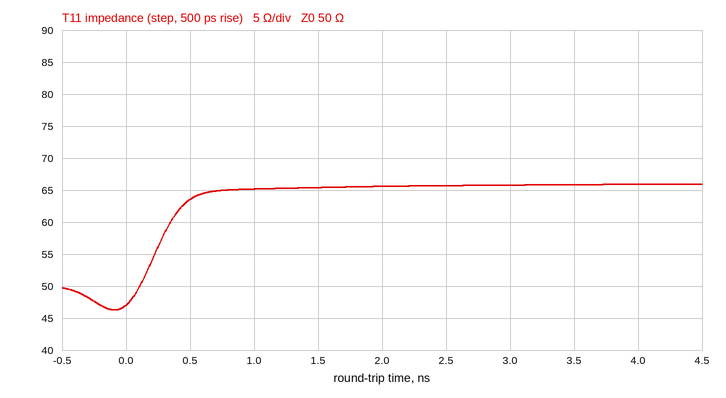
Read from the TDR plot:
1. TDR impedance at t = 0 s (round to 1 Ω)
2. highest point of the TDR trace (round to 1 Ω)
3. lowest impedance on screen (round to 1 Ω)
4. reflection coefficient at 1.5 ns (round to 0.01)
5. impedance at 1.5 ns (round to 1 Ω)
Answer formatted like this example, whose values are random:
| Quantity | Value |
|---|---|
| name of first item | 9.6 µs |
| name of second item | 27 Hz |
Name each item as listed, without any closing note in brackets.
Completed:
| Quantity | Value |
|---|---|
| TDR impedance at t = 0 s | 47 Ω |
| highest point of the TDR trace | 66 Ω |
| lowest impedance on screen | 46 Ω |
| reflection coefficient at 1.5 ns | +0.13 |
| impedance at 1.5 ns | 65 Ω |
